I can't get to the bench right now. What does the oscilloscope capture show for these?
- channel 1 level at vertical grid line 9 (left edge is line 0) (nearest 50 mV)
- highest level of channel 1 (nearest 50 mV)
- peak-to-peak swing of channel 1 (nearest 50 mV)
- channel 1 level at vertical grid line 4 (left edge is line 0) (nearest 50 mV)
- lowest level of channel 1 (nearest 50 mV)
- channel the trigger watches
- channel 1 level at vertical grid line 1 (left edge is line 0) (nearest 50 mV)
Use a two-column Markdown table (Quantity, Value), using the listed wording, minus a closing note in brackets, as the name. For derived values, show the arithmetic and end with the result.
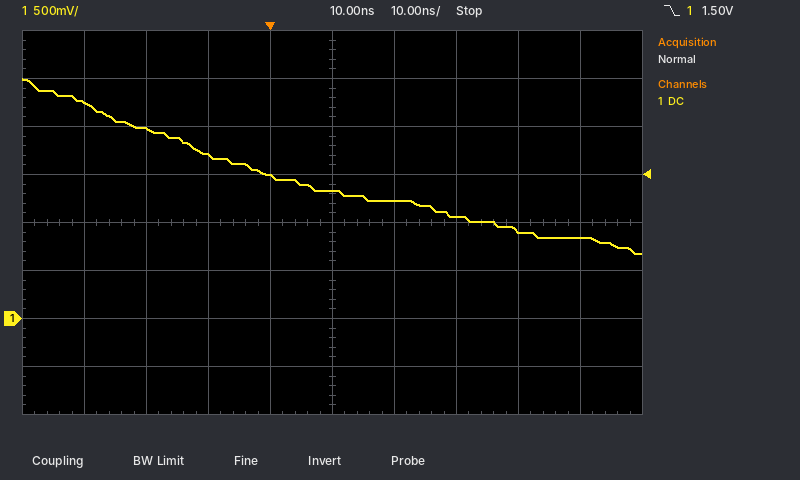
| Quantity | Value |
|---|---|
| channel 1 level at vertical grid line 9 (left edge is line 0) | 850 mV |
| highest level of channel 1 | 2.50 V |
| peak-to-peak swing of channel 1 | 2.50 V − (700 mV) = 1.80 V |
| channel 1 level at vertical grid line 4 (left edge is line 0) | 1.50 V |
| lowest level of channel 1 | 700 mV |
| channel the trigger watches | channel 1 |
| channel 1 level at vertical grid line 1 (left edge is line 0) | 2.25 V |
